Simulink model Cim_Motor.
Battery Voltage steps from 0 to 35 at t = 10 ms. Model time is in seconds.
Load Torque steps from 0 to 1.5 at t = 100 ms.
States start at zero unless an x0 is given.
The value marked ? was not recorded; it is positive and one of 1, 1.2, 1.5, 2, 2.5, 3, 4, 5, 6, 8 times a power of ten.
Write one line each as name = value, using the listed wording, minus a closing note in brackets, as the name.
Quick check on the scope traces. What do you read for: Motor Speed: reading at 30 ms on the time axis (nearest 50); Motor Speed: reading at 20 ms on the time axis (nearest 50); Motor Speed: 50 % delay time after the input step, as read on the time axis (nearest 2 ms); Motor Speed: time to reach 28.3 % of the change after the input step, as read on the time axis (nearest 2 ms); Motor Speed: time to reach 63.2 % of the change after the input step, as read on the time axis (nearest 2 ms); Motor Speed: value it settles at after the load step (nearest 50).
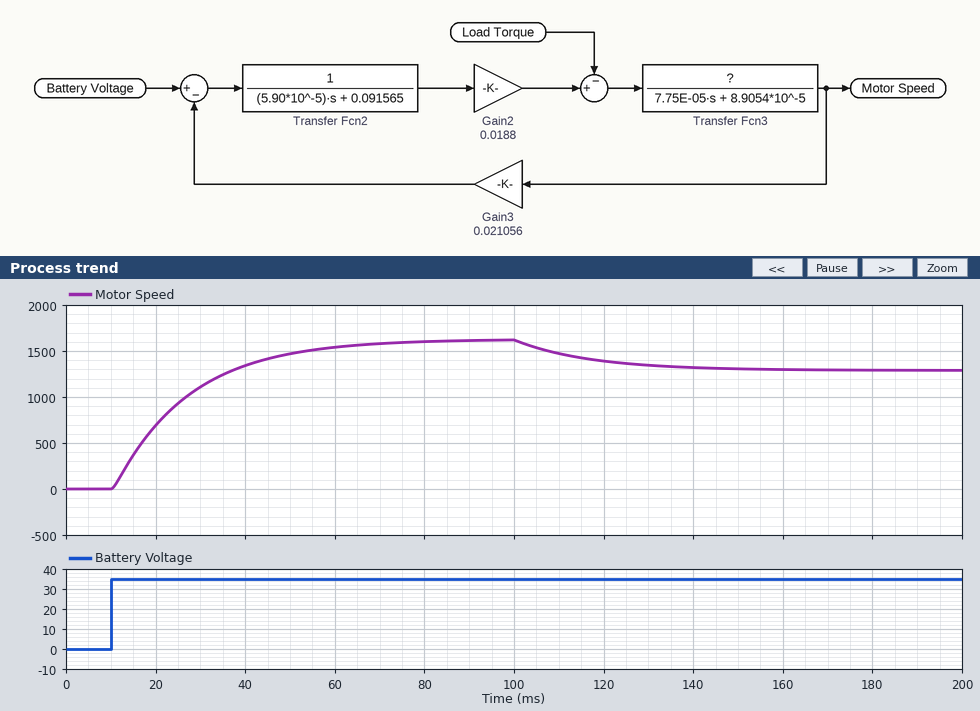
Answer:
Motor Speed: reading at 30 ms on the time axis = 1100
Motor Speed: reading at 20 ms on the time axis = 700
Motor Speed: 50 % delay time after the input step, as read on the time axis = 22 ms
Motor Speed: time to reach 28.3 % of the change after the input step, as read on the time axis = 16 ms
Motor Speed: time to reach 63.2 % of the change after the input step, as read on the time axis = 28 ms
Motor Speed: value it settles at after the load step = 1300
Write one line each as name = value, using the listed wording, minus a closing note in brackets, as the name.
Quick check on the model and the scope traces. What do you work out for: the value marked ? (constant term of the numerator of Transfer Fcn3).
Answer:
the value marked ? = 1
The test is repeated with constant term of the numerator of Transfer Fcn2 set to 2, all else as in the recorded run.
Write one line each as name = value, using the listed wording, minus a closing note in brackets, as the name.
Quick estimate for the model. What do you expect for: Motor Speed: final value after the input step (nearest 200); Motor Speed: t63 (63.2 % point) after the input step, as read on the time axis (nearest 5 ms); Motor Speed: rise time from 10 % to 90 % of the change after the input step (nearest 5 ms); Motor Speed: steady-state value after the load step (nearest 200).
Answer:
Motor Speed: final value after the input step = 1600
Motor Speed: t63 (63.2 % point) after the input step, as read on the time axis = 20 ms
Motor Speed: rise time from 10 % to 90 % of the change after the input step = 20 ms
Motor Speed: steady-state value after the load step = 1400
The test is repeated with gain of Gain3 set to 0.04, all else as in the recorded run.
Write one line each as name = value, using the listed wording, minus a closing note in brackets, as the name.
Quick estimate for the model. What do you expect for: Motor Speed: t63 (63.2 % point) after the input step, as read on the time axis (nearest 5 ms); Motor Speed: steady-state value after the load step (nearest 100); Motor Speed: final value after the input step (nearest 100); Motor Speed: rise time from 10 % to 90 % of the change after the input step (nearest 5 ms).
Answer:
Motor Speed: t63 (63.2 % point) after the input step, as read on the time axis = 20 ms
Motor Speed: steady-state value after the load step = 700
Motor Speed: final value after the input step = 900
Motor Speed: rise time from 10 % to 90 % of the change after the input step = 20 ms
